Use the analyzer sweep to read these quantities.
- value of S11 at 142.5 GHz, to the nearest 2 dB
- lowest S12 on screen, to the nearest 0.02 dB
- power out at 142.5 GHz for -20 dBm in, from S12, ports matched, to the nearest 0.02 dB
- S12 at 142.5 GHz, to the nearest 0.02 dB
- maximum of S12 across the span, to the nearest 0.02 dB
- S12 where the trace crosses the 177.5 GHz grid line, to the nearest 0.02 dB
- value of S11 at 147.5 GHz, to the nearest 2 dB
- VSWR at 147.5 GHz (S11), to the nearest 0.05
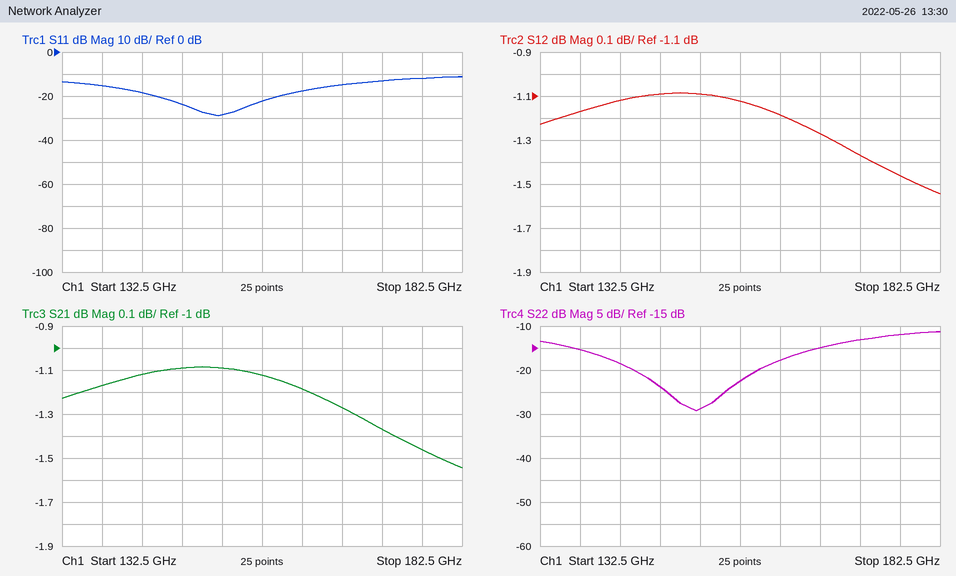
-18 dB
-1.54 dB
-21.12 dBm
-1.12 dB
-1.08 dB
-1.46 dB
-24 dB
1.15
